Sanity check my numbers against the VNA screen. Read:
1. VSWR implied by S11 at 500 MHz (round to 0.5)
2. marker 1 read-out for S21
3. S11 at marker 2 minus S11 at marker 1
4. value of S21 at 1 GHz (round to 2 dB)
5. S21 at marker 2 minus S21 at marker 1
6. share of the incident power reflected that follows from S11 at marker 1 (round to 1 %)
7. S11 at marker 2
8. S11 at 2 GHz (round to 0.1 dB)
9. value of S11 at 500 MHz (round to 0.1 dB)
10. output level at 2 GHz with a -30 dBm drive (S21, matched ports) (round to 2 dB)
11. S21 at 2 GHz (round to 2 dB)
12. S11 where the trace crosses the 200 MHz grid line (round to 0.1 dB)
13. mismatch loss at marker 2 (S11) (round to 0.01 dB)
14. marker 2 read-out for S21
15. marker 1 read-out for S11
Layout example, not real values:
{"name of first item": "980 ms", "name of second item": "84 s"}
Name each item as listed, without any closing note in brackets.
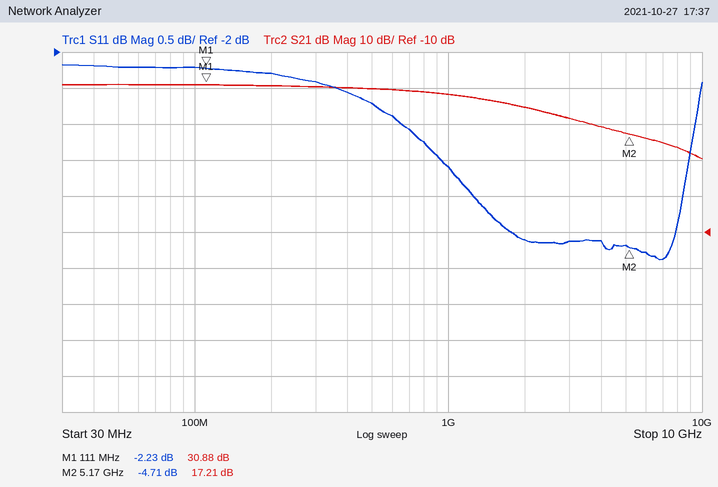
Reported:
{"VSWR implied by S11 at 500 MHz": "6.5", "marker 1 read-out for S21": "30.88 dB", "S11 at marker 2 minus S11 at marker 1": "-2.48 dB", "value of S21 at 1 GHz": "28 dB", "S21 at marker 2 minus S21 at marker 1": "-13.67 dB", "share of the incident power reflected that follows from S11 at marker 1": "60 %", "S11 at marker 2": "-4.71 dB", "S11 at 2 GHz": "-4.6 dB", "value of S11 at 500 MHz": "-2.7 dB", "output level at 2 GHz with a -30 dBm drive (S21, matched ports)": "-6 dBm", "S21 at 2 GHz": "24 dB", "S11 where the trace crosses the 200 MHz grid line": "-2.3 dB", "mismatch loss at marker 2 (S11)": "1.79 dB", "marker 2 read-out for S21": "17.21 dB", "marker 1 read-out for S11": "-2.23 dB"}
